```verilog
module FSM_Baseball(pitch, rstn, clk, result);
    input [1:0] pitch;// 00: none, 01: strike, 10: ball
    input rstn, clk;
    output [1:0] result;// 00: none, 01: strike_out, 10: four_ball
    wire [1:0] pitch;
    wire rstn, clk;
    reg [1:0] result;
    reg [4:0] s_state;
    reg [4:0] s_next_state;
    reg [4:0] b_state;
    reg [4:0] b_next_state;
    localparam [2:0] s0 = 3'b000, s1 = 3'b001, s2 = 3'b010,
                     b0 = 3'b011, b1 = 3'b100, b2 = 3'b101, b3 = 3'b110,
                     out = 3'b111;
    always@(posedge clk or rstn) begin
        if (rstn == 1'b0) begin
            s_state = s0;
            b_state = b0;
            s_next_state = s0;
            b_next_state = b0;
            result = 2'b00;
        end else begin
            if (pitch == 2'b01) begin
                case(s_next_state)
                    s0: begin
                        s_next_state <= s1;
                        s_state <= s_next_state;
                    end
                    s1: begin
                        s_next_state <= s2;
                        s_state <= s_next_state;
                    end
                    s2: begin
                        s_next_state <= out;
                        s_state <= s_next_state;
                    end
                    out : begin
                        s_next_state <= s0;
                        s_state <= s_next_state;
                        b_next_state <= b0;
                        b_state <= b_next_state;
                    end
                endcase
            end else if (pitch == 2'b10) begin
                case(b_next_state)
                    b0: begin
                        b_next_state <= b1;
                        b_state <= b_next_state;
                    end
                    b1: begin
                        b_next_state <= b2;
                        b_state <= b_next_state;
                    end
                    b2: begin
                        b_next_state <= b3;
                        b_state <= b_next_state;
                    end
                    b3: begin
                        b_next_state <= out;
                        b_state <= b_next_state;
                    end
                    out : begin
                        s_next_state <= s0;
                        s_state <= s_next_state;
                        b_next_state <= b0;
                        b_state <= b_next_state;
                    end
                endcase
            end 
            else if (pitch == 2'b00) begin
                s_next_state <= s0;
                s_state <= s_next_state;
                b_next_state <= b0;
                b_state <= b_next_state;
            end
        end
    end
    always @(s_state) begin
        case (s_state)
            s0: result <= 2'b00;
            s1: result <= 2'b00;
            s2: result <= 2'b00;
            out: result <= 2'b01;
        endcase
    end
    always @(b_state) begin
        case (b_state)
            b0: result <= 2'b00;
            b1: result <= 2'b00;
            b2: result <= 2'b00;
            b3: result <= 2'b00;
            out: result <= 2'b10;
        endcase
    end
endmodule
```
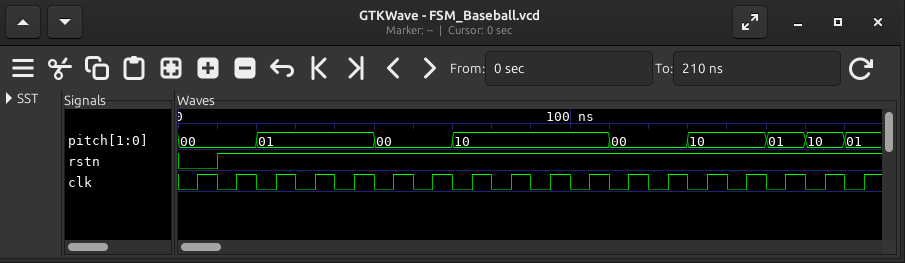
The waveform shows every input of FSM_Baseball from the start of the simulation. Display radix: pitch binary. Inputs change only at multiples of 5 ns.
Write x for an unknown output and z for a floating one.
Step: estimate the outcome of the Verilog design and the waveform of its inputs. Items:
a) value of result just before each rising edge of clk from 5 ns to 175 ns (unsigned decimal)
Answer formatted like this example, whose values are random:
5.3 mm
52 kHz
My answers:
0, 0, 0, 0, 0, 0, 1, 0, 0, 0, 0, 0, 2, 0, 0, 0, 0, 0
